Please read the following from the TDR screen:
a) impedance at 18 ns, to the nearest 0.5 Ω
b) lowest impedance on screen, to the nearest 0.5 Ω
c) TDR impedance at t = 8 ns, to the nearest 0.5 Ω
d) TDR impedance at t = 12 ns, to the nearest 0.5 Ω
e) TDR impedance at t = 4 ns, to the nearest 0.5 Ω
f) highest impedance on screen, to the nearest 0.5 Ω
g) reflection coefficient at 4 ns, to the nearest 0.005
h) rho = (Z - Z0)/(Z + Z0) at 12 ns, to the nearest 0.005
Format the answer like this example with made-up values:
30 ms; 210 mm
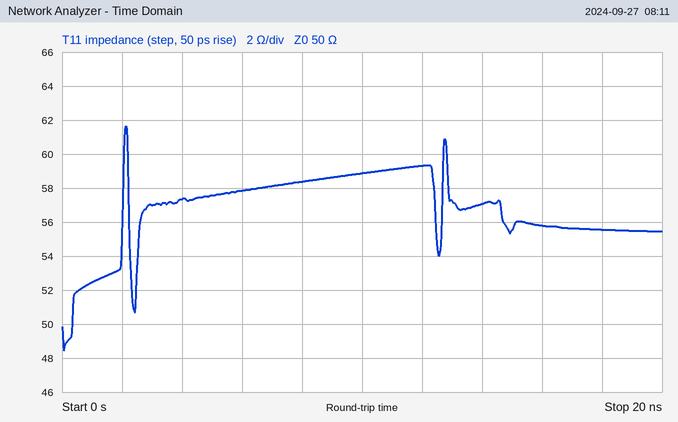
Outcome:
55.5 Ω; 48.5 Ω; 58.5 Ω; 59.5 Ω; 57.5 Ω; 61.5 Ω; +0.070; +0.085
